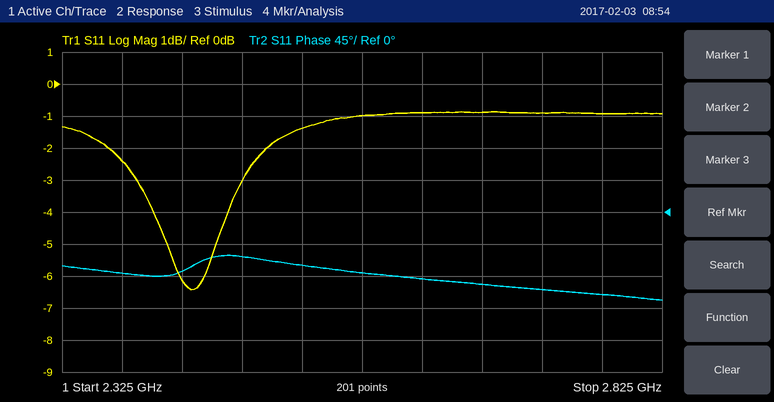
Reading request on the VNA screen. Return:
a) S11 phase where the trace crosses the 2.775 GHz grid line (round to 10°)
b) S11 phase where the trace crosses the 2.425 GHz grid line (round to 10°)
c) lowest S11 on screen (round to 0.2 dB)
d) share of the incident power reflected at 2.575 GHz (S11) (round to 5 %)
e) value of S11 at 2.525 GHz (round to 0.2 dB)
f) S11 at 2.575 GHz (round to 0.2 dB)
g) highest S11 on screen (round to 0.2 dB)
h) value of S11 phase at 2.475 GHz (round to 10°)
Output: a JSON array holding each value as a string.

["-120°", "-80°", "-6.4 dB", "80 %", "-1.4 dB", "-1.0 dB", "-0.8 dB", "-60°"]
